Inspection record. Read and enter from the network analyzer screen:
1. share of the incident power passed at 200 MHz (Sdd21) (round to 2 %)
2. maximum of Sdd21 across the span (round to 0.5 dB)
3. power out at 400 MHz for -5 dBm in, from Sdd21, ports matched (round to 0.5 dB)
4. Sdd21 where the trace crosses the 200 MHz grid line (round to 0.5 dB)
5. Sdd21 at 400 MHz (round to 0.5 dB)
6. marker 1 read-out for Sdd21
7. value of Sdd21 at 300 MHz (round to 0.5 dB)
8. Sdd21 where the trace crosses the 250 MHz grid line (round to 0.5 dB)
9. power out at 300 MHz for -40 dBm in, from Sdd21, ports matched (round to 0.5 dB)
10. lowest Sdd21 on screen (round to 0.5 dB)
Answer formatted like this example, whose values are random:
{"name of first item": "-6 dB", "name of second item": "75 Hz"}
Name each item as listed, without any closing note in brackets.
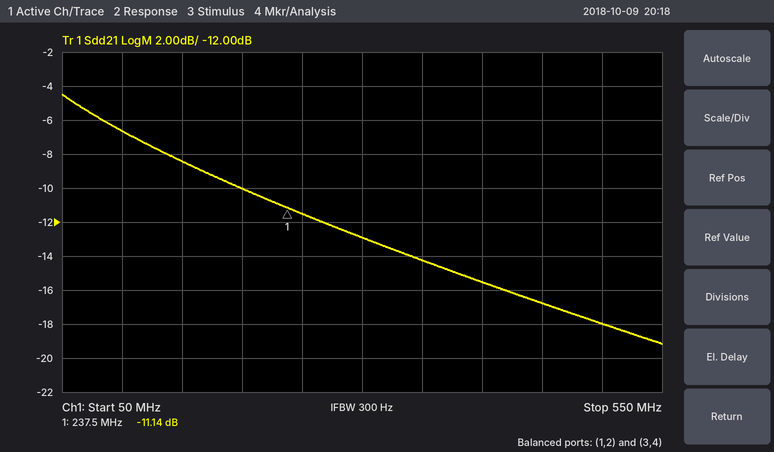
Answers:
{"share of the incident power passed at 200 MHz (Sdd21)": "10 %", "maximum of Sdd21 across the span": "-4.5 dB", "power out at 400 MHz for -5 dBm in, from Sdd21, ports matched": "-20.5 dBm", "Sdd21 where the trace crosses the 200 MHz grid line": "-10.0 dB", "Sdd21 at 400 MHz": "-15.5 dB", "marker 1 read-out for Sdd21": "-11.14 dB", "value of Sdd21 at 300 MHz": "-13.0 dB", "Sdd21 where the trace crosses the 250 MHz grid line": "-11.5 dB", "power out at 300 MHz for -40 dBm in, from Sdd21, ports matched": "-53.0 dBm", "lowest Sdd21 on screen": "-19.0 dB"}
